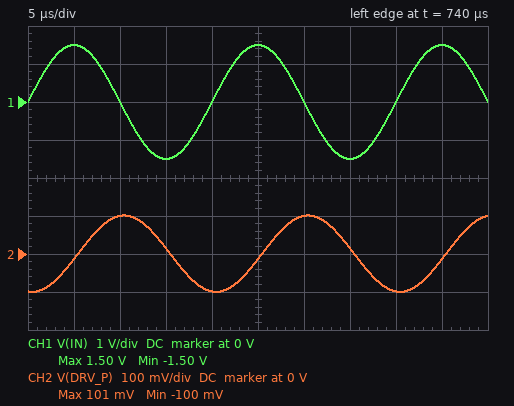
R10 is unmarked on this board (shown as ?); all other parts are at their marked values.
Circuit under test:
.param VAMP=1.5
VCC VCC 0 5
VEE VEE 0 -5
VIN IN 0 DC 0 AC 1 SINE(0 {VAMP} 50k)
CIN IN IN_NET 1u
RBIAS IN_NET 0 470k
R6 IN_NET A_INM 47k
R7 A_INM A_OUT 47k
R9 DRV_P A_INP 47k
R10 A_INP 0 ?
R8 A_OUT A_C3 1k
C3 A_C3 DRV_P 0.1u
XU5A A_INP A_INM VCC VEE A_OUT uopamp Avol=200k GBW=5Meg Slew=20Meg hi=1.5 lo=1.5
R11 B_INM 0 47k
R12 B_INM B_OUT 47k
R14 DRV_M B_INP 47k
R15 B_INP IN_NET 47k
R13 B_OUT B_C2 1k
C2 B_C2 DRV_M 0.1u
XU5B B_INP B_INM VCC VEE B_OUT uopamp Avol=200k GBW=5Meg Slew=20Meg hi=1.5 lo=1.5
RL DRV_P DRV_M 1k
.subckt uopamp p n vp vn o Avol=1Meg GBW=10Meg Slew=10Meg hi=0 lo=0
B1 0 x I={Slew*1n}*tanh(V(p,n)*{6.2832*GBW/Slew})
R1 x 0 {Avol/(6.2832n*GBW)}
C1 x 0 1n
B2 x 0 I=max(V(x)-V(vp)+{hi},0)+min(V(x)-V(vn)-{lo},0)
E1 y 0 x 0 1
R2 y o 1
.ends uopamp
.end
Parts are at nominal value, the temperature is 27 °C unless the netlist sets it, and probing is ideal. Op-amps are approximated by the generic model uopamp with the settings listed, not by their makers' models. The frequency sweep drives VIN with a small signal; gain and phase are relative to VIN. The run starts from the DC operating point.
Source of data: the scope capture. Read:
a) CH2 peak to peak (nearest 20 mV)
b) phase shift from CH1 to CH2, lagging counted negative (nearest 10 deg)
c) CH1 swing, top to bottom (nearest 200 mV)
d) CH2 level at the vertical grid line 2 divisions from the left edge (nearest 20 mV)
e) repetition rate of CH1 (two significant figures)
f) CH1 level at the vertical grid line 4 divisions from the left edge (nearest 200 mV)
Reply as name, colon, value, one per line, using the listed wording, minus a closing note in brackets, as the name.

CH2 peak to peak: 200 mV
phase shift from CH1 to CH2, lagging counted negative: -100 deg
CH1 swing, top to bottom: 3.0 V
CH2 level at the vertical grid line 2 divisions from the left edge: 100 mV
repetition rate of CH1: 50 kHz
CH1 level at the vertical grid line 4 divisions from the left edge: 0 V
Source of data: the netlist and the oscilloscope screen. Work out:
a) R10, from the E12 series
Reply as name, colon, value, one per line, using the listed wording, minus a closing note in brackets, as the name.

R10, from the E12 series: 27 kΩ
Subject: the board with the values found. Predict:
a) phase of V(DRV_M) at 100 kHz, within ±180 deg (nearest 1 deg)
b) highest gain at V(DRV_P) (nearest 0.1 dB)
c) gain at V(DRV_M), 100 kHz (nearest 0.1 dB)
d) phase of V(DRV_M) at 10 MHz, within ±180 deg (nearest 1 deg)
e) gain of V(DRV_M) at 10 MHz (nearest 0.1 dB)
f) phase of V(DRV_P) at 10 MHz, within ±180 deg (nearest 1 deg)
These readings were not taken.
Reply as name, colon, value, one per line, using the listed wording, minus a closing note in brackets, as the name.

phase of V(DRV_M) at 100 kHz, within ±180 deg: -11 deg
highest gain at V(DRV_P): -7.5 dB
gain at V(DRV_M), 100 kHz: -0.3 dB
phase of V(DRV_M) at 10 MHz, within ±180 deg: -77 deg
gain of V(DRV_M) at 10 MHz: -21.5 dB
phase of V(DRV_P) at 10 MHz, within ±180 deg: 100 deg
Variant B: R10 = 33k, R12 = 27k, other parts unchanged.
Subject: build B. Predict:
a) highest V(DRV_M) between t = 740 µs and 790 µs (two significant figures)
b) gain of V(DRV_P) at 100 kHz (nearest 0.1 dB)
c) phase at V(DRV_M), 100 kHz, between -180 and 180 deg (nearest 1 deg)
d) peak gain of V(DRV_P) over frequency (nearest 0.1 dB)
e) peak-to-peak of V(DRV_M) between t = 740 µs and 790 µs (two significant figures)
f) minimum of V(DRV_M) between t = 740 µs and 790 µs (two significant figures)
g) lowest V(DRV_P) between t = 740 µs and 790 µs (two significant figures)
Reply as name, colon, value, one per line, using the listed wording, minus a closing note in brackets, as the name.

highest V(DRV_M) between t = 740 µs and 790 µs: 190 mV
gain of V(DRV_P) at 100 kHz: -0.7 dB
phase at V(DRV_M), 100 kHz, between -180 and 180 deg: 134 deg
peak gain of V(DRV_P) over frequency: -0.6 dB
peak-to-peak of V(DRV_M) between t = 740 µs and 790 µs: 380 mV
minimum of V(DRV_M) between t = 740 µs and 790 µs: -190 mV
lowest V(DRV_P) between t = 740 µs and 790 µs: -1.4 V
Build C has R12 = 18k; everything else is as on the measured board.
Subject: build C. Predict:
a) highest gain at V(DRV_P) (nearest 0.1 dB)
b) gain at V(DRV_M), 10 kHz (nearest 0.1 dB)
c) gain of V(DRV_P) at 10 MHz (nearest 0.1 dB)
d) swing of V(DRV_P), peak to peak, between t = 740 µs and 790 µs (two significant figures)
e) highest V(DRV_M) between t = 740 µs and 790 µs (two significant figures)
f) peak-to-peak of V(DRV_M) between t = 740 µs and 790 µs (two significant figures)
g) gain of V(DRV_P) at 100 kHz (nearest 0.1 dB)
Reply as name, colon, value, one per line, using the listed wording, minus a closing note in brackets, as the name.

highest gain at V(DRV_P): -1.0 dB
gain at V(DRV_M), 10 kHz: -16.1 dB
gain of V(DRV_P) at 10 MHz: -21.8 dB
swing of V(DRV_P), peak to peak, between t = 740 µs and 790 µs: 2.7 V
highest V(DRV_M) between t = 740 µs and 790 µs: 220 mV
peak-to-peak of V(DRV_M) between t = 740 µs and 790 µs: 440 mV
gain of V(DRV_P) at 100 kHz: -1.1 dB
